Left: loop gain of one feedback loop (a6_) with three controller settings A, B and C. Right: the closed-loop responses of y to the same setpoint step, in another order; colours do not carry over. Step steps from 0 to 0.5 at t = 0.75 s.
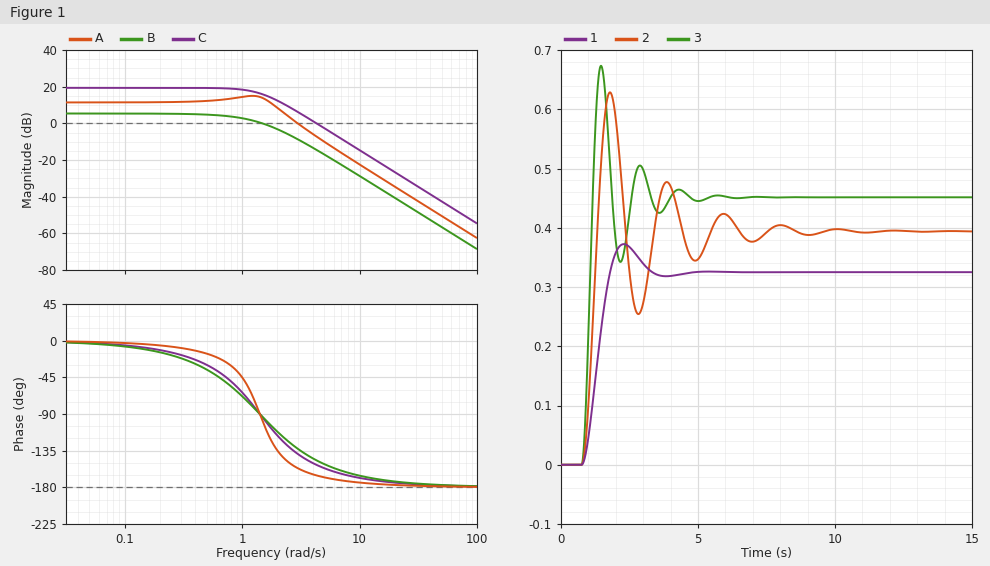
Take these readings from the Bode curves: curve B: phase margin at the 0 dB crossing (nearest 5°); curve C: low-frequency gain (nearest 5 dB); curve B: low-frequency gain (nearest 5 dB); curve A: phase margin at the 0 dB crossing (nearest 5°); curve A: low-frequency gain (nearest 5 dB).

85°
20 dB
5 dB
25°
10 dB
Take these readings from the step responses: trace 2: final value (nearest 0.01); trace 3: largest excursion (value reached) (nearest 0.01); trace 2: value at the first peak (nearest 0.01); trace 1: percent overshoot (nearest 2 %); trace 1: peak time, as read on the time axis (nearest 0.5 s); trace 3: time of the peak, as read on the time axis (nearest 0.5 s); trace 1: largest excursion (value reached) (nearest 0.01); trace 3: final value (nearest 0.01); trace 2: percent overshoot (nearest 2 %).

0.39
0.67
0.63
14 %
2.5 s
1.5 s
0.37
0.45
60 %
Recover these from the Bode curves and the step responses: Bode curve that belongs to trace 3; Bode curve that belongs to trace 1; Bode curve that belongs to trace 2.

C
B
A
